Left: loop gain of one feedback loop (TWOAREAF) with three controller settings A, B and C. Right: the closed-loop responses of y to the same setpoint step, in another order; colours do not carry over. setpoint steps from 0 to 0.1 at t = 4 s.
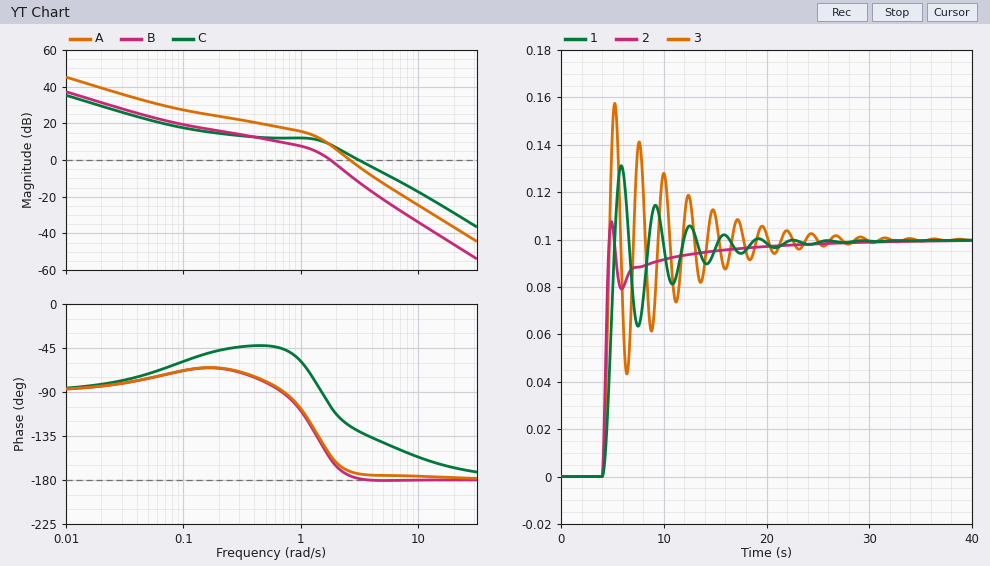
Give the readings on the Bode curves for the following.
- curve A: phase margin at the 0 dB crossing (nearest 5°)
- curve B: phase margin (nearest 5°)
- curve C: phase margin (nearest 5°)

10°
20°
50°
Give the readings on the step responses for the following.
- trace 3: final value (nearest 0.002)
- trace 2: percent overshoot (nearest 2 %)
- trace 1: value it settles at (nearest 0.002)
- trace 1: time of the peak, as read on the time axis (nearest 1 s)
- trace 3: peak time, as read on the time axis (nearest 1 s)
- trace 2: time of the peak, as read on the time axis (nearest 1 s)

0.100
8 %
0.100
6 s
5 s
5 s
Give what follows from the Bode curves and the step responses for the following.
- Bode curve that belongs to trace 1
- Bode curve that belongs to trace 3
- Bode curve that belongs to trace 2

B
A
C
